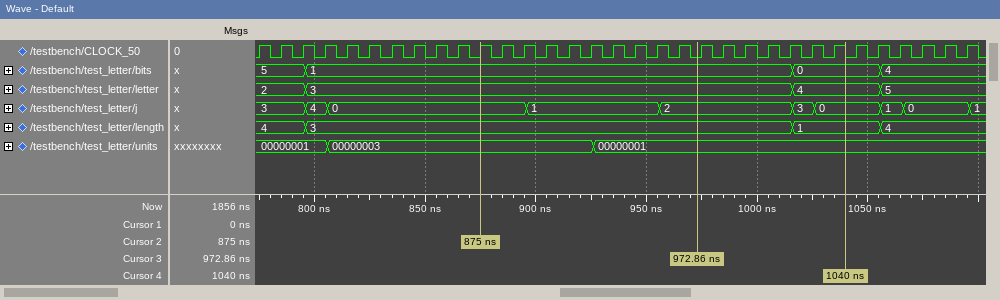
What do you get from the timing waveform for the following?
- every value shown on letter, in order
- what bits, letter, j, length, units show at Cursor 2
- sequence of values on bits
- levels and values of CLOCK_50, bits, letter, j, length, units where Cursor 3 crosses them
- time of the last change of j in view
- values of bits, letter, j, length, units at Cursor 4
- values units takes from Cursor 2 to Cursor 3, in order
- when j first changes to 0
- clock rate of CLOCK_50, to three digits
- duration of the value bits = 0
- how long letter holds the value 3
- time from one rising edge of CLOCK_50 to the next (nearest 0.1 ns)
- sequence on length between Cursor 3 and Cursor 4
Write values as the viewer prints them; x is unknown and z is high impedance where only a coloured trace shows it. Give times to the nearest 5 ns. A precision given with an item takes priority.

2, 3, 4, 5
bits=1, letter=3, j=0, length=3, units=00000003
5, 1, 0, 4
CLOCK_50=0, bits=1, letter=3, j=2, length=3, units=00000001
1095 ns
bits=0, letter=4, j=0, length=1, units=00000001
00000003, 00000001
805 ns
100 MHz
40 ns
220 ns
10 ns
3, 1
